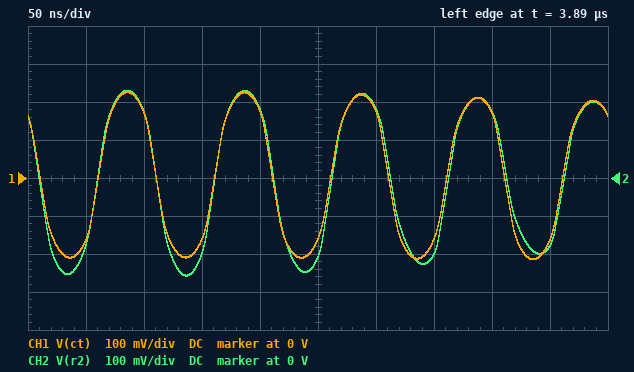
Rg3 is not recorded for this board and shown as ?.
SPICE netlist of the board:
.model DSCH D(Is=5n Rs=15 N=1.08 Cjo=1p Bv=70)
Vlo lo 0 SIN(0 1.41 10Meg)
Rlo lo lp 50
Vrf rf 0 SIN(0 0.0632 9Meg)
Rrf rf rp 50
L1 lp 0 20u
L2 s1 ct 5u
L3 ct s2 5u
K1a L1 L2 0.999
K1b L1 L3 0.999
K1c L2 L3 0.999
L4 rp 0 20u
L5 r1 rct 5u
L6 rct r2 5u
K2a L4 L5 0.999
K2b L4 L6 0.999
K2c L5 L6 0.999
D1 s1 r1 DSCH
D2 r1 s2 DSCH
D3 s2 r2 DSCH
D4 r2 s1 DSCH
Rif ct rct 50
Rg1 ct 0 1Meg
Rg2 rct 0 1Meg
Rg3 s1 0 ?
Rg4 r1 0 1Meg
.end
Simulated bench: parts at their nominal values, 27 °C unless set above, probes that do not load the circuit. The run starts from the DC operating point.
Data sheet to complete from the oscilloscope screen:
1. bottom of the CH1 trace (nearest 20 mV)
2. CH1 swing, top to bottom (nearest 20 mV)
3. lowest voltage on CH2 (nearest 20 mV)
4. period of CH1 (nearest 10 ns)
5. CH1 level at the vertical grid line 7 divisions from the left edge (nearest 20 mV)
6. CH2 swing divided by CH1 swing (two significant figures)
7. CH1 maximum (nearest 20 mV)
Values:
-220 mV
440 mV
-260 mV
100 ns
-160 mV
1.1
220 mV
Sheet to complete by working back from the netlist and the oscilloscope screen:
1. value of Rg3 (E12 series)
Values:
470 kΩ
